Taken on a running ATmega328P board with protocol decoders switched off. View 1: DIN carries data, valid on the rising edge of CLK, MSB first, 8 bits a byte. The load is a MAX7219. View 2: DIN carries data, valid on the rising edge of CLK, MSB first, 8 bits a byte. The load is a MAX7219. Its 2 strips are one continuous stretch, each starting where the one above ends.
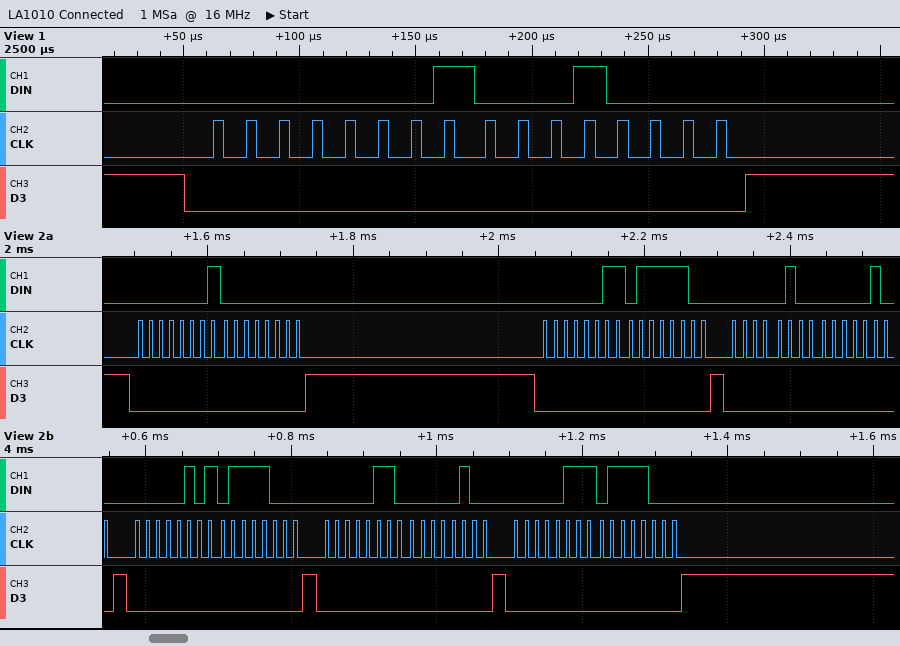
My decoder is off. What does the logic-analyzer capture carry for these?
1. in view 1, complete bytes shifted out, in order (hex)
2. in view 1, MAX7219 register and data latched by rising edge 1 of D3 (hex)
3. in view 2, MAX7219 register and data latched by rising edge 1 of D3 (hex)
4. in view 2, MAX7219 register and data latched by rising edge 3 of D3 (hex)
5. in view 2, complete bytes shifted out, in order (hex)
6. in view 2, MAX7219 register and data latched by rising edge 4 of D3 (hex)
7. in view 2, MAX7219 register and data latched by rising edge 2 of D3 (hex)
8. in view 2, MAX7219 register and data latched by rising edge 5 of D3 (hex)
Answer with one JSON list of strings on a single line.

["01 10", "register 0x1, data 0x10", "register 0x1, data 0x00", "register 0x4, data 0x04", "0x01 0x00 0x03 0x7C 0x04 0x04 0x05 0x78 0x06 0x04 0x07 0x78", "register 0x5, data 0x78", "register 0x3, data 0x7C", "register 0x6, data 0x04"]
